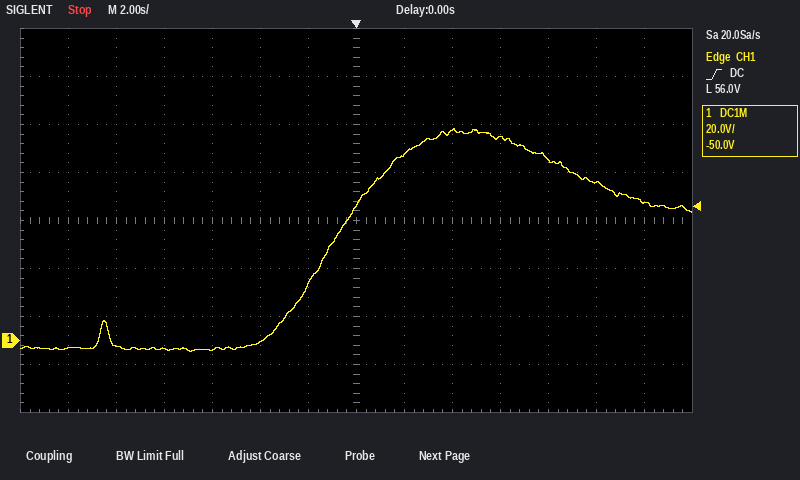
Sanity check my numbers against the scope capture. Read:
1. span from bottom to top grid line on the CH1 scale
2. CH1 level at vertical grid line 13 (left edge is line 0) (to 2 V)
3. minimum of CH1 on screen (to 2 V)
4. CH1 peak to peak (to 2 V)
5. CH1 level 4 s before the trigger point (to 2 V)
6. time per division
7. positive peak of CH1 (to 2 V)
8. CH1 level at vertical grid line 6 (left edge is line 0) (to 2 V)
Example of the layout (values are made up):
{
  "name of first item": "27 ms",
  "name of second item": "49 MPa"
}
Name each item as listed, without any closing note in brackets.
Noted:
{
  "span from bottom to top grid line on the CH1 scale": "160 V",
  "CH1 level at vertical grid line 13 (left edge is line 0)": "58 V",
  "minimum of CH1 on screen": "-4 V",
  "CH1 peak to peak": "92 V",
  "CH1 level 4 s before the trigger point": "0 V",
  "time per division": "2 s",
  "positive peak of CH1": "88 V",
  "CH1 level at vertical grid line 6 (left edge is line 0)": "24 V"
}
